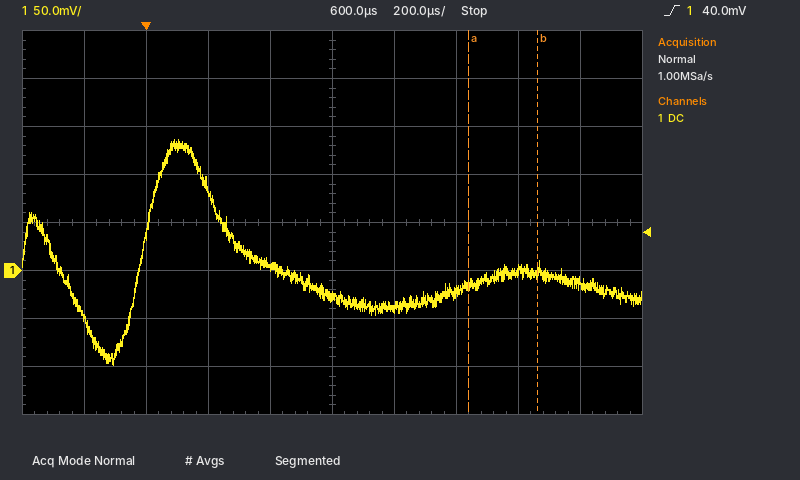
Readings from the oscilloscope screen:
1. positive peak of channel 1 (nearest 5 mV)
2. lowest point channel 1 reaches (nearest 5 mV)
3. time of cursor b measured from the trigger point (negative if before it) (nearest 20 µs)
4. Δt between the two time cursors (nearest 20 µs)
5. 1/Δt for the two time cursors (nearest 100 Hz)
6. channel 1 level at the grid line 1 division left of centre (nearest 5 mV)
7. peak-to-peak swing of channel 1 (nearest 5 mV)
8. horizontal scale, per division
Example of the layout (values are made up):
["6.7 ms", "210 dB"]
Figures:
["135 mV", "-100 mV", "+1.26 ms", "220 µs", "4.5 kHz", "5 mV", "235 mV", "200 µs"]
